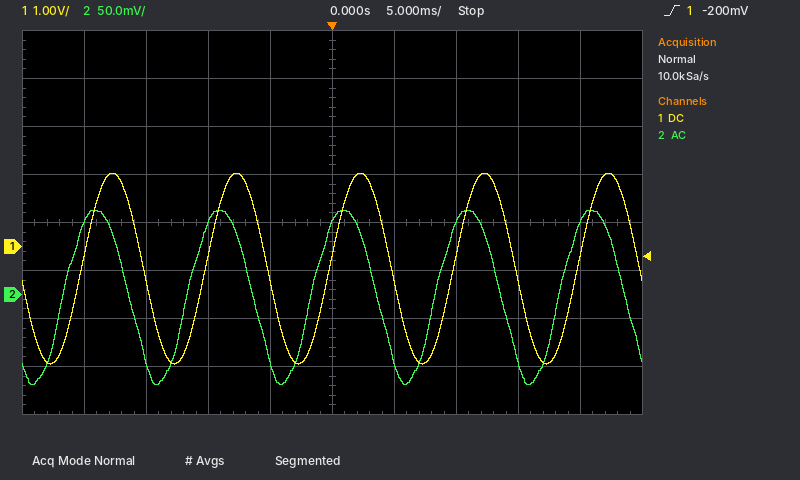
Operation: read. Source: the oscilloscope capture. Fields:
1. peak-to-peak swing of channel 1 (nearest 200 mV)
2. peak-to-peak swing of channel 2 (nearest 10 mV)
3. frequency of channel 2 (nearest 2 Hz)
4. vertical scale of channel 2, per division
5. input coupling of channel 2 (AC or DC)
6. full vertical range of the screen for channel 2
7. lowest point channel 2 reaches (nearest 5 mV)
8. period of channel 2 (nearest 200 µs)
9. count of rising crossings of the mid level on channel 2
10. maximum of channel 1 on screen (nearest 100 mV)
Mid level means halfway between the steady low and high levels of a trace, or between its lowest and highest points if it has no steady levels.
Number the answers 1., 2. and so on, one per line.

1. 4.0 V
2. 180 mV
3. 100 Hz
4. 50 mV
5. AC
6. 400 mV
7. -95 mV
8. 10.0 ms
9. 5
10. 1.5 V
